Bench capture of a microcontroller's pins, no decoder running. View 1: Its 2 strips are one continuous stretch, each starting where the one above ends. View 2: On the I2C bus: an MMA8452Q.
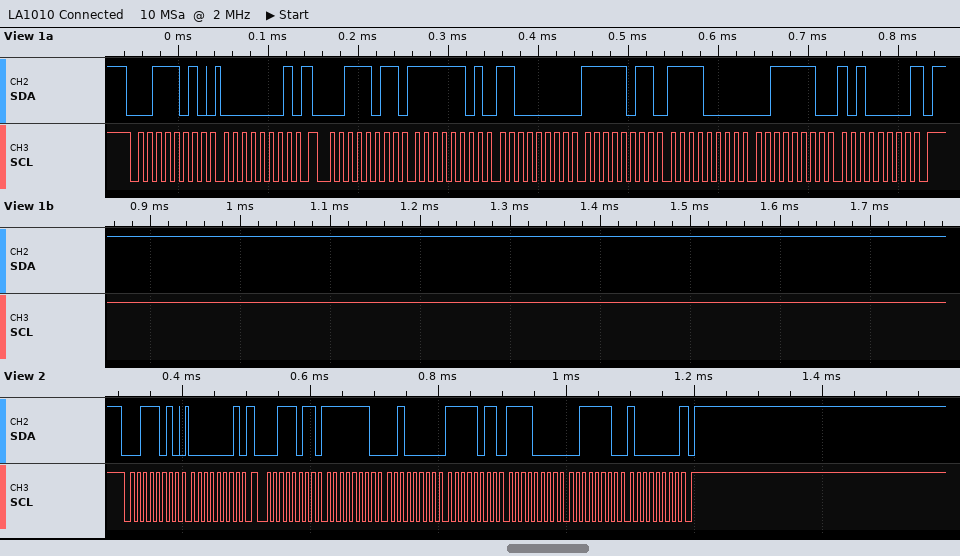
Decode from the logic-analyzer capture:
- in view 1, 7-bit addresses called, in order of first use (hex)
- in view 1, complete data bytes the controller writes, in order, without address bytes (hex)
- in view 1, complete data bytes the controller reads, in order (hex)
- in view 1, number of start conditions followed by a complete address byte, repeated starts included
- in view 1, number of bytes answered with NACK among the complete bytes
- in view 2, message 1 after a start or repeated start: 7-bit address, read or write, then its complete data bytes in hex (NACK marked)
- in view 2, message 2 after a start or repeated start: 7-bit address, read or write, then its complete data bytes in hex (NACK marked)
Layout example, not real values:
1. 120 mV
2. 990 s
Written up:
1. 0x1D
2. 01
3. FD C0 FB F0 3E A0
4. 2
5. 1
6. 0x1D write: 01
7. 0x1D read: FE 20 FB F0 3E 80 NACK
